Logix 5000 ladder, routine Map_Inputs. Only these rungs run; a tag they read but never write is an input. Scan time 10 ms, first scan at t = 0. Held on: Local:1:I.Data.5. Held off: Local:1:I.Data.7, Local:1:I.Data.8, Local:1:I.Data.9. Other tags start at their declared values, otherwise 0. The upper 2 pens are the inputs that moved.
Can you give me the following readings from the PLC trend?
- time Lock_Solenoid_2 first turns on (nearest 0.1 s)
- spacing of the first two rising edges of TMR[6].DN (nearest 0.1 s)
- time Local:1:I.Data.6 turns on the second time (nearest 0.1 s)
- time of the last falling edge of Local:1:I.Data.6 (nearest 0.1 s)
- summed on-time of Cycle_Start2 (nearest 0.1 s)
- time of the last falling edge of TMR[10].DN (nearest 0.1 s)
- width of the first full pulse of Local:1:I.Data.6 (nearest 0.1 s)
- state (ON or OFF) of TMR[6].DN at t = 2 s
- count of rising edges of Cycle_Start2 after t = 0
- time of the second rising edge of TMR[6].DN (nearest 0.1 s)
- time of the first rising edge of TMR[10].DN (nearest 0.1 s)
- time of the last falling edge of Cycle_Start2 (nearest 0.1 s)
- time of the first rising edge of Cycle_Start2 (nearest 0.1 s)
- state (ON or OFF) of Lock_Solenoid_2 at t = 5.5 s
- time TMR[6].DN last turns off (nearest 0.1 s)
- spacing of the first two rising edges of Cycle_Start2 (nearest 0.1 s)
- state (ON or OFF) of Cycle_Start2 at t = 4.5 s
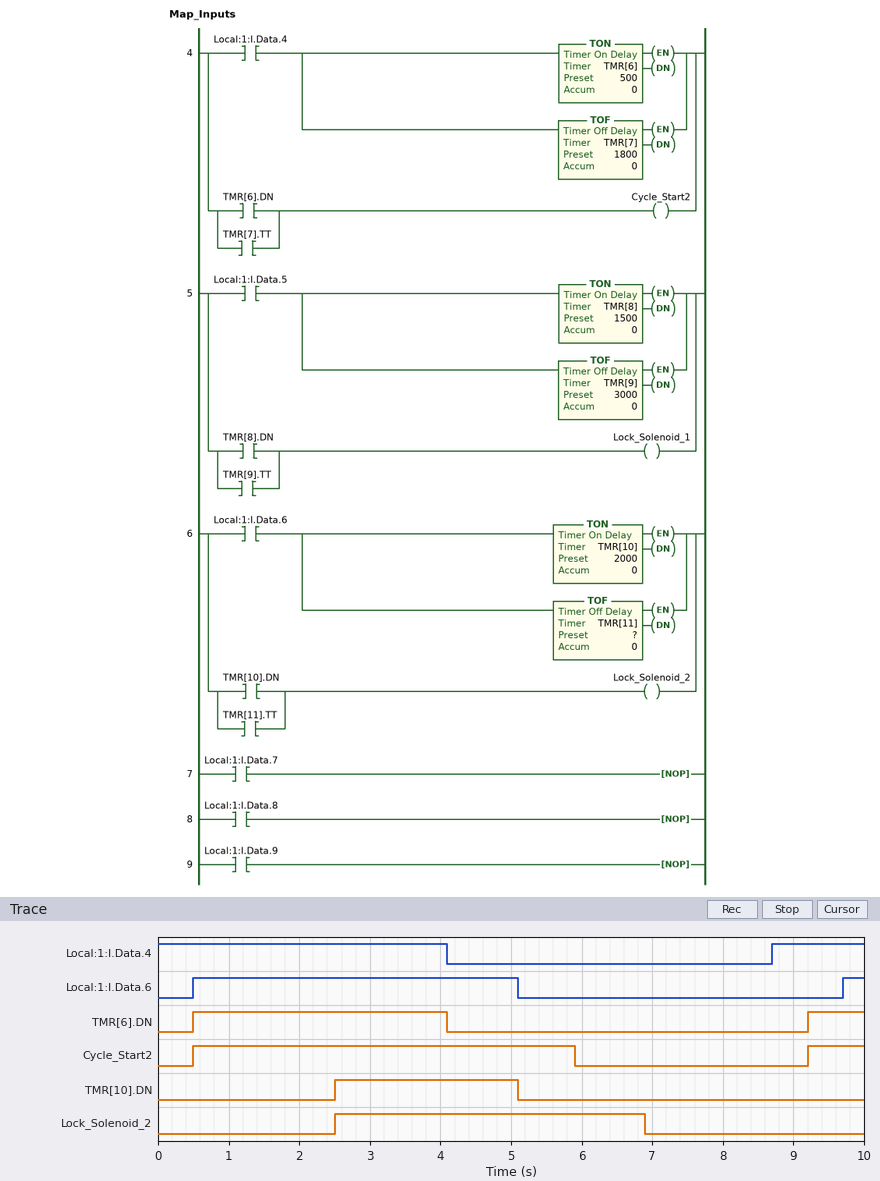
2.5 s
8.7 s
9.7 s
5.1 s
6.2 s
5.1 s
4.6 s
ON
2
9.2 s
2.5 s
5.9 s
0.5 s
ON
4.1 s
8.7 s
ON
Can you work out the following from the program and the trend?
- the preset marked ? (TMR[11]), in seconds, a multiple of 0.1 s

1.8 s
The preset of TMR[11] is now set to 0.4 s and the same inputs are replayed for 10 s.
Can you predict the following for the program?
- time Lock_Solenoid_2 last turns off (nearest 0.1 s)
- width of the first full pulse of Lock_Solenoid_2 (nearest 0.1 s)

5.5 s
3.0 s
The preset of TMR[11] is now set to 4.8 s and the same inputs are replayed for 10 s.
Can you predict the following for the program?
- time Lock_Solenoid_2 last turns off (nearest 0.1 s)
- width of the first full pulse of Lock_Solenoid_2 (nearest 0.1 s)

9.7 s
7.2 s
